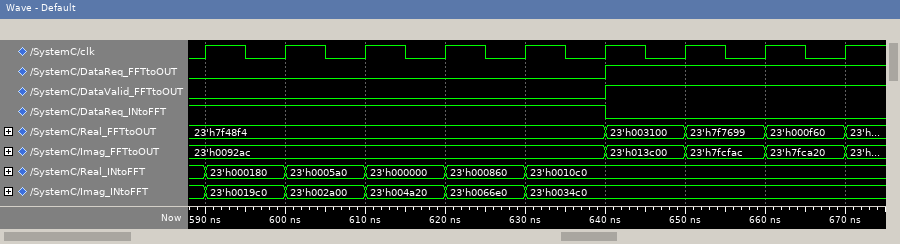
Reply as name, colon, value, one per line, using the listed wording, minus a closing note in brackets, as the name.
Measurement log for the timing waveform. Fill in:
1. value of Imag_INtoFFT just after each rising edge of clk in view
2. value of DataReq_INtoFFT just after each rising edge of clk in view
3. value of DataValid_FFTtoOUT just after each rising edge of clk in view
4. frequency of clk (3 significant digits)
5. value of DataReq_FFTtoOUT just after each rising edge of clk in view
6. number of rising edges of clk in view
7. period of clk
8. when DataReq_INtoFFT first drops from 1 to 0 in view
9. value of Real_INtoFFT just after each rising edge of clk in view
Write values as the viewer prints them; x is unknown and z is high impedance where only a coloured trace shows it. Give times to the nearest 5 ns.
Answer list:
value of Imag_INtoFFT just after each rising edge of clk in view: 23'h0019c0, 23'h002a00, 23'h004a20, 23'h0066e0, 23'h0034c0, 23'h0034c0, 23'h0034c0, 23'h0034c0, 23'h0034c0
value of DataReq_INtoFFT just after each rising edge of clk in view: 1 1 1 1 1 0 0 0 0
value of DataValid_FFTtoOUT just after each rising edge of clk in view: 0 0 0 0 0 1 1 1 1
frequency of clk: 100 MHz
value of DataReq_FFTtoOUT just after each rising edge of clk in view: 0 0 0 0 0 1 1 1 1
number of rising edges of clk in view: 9
period of clk: 10 ns
when DataReq_INtoFFT first drops from 1 to 0 in view: 640 ns
value of Real_INtoFFT just after each rising edge of clk in view: 23'h000180, 23'h0005a0, 23'h000000, 23'h000860, 23'h0010c0, 23'h0010c0, 23'h0010c0, 23'h0010c0, 23'h0010c0
